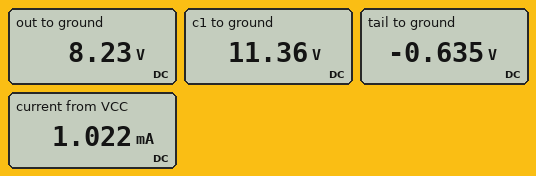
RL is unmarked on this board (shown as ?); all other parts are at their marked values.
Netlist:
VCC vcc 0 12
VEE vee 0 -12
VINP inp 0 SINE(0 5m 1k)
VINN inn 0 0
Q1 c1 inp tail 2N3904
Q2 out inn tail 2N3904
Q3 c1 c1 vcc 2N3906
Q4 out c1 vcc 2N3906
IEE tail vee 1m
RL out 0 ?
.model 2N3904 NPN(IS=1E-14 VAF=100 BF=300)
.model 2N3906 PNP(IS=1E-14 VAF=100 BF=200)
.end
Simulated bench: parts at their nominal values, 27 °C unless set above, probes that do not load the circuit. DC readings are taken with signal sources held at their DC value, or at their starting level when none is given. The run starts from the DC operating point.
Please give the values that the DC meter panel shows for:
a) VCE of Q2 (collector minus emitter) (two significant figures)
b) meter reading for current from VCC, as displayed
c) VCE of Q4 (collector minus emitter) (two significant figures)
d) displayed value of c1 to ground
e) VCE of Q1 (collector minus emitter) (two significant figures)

8.9 V
1.022 mA
-3.8 V
11.36 V
12 V
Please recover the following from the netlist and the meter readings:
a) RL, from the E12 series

330 kΩ
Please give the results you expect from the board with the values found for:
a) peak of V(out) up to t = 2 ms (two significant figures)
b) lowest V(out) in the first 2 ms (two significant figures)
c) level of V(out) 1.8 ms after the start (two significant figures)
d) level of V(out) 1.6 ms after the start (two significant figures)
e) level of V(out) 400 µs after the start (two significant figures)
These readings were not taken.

12 V
490 mV
870 mV
3.7 V
12 V
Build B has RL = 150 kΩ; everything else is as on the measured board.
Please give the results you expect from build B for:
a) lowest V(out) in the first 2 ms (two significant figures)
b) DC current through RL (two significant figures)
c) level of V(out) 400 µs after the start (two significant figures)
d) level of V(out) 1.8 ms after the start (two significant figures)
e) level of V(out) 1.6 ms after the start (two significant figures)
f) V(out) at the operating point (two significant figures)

380 mV
43 µA
9.9 V
680 mV
2.9 V
6.4 V
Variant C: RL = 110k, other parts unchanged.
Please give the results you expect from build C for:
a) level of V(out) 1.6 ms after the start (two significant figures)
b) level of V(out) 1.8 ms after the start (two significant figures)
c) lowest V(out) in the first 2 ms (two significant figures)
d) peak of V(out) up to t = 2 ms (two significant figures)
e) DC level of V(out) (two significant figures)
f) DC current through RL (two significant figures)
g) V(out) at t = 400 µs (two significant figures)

2.5 V
590 mV
330 mV
11 V
5.6 V
51 µA
8.6 V
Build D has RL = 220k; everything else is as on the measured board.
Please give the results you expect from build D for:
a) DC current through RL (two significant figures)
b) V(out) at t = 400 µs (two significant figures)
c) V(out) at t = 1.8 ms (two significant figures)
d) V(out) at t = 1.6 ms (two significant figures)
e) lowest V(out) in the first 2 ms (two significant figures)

33 µA
11 V
780 mV
3.3 V
440 mV
